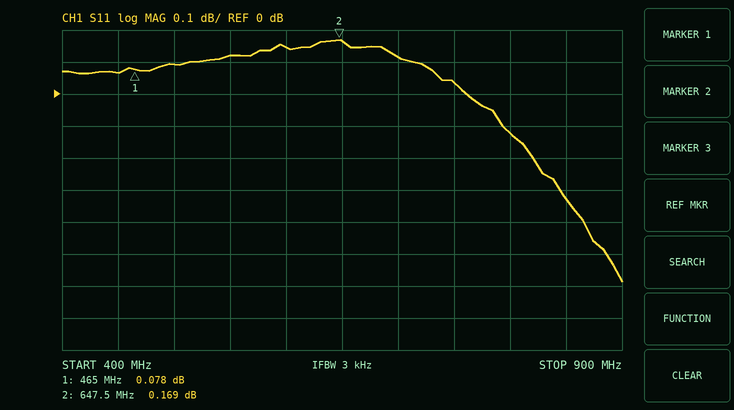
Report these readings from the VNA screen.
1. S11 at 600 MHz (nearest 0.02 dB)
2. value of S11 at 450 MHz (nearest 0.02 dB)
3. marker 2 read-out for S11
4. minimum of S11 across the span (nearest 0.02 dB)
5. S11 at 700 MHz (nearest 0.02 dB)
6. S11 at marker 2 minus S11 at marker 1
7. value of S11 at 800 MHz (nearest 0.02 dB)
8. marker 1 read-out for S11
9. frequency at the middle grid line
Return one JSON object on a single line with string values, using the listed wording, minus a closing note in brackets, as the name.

{"S11 at 600 MHz": "0.14 dB", "value of S11 at 450 MHz": "0.06 dB", "marker 2 read-out for S11": "0.169 dB", "minimum of S11 across the span": "-0.58 dB", "S11 at 700 MHz": "0.12 dB", "S11 at marker 2 minus S11 at marker 1": "0.091 dB", "value of S11 at 800 MHz": "-0.12 dB", "marker 1 read-out for S11": "0.078 dB", "frequency at the middle grid line": "650 MHz"}
